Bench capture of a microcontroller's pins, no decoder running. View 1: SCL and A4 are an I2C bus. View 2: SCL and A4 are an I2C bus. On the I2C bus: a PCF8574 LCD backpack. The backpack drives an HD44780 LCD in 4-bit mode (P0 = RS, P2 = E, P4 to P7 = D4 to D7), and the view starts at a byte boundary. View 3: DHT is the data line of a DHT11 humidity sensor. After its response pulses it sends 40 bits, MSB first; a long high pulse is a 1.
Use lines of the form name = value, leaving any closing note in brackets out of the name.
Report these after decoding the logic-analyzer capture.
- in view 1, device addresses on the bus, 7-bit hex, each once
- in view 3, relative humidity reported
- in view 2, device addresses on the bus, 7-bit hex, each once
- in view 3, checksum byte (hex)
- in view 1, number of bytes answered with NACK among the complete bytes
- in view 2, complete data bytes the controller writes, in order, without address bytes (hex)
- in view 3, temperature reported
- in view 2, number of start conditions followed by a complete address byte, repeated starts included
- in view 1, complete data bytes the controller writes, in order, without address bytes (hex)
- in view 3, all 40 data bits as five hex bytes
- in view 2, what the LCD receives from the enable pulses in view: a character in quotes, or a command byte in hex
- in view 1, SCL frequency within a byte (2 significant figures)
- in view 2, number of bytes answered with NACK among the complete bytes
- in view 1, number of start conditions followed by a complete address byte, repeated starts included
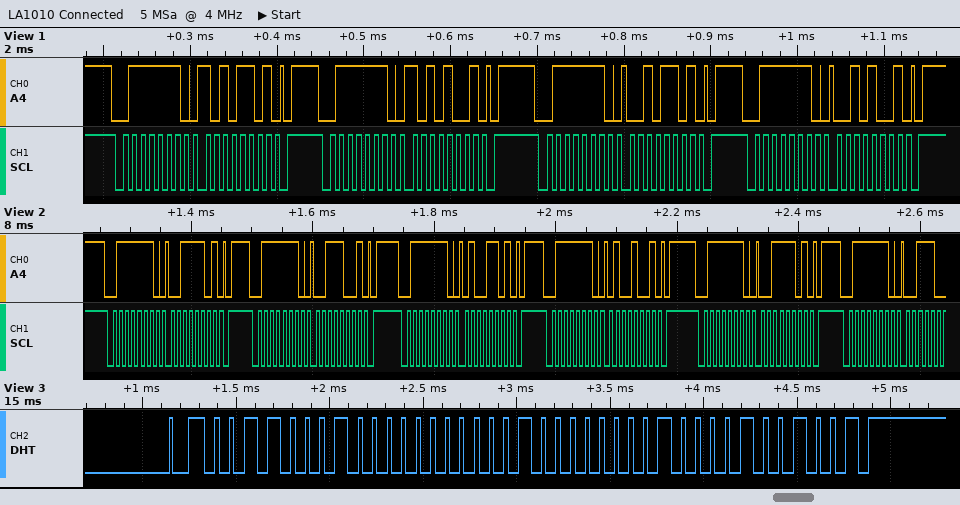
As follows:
in view 1, device addresses on the bus, 7-bit hex, each once = 0x3F
in view 3, relative humidity reported = 49 %
in view 2, device addresses on the bus, 7-bit hex, each once = 0x3F
in view 3, checksum byte = 0x49
in view 1, number of bytes answered with NACK among the complete bytes = 0
in view 2, complete data bytes the controller writes, in order, without address bytes = 3D 39 4D 49 3D
in view 3, temperature reported = 16.8 °C
in view 2, number of start conditions followed by a complete address byte, repeated starts included = 6
in view 1, complete data bytes the controller writes, in order, without address bytes = AD A9 2D 29
in view 3, all 40 data bits as five hex bytes = 31 00 10 08 49
in view 2, what the LCD receives from the enable pulses in view: a character in quotes, or a command byte in hex = '4'
in view 1, SCL frequency within a byte = 100 kHz
in view 2, number of bytes answered with NACK among the complete bytes = 0
in view 1, number of start conditions followed by a complete address byte, repeated starts included = 4
